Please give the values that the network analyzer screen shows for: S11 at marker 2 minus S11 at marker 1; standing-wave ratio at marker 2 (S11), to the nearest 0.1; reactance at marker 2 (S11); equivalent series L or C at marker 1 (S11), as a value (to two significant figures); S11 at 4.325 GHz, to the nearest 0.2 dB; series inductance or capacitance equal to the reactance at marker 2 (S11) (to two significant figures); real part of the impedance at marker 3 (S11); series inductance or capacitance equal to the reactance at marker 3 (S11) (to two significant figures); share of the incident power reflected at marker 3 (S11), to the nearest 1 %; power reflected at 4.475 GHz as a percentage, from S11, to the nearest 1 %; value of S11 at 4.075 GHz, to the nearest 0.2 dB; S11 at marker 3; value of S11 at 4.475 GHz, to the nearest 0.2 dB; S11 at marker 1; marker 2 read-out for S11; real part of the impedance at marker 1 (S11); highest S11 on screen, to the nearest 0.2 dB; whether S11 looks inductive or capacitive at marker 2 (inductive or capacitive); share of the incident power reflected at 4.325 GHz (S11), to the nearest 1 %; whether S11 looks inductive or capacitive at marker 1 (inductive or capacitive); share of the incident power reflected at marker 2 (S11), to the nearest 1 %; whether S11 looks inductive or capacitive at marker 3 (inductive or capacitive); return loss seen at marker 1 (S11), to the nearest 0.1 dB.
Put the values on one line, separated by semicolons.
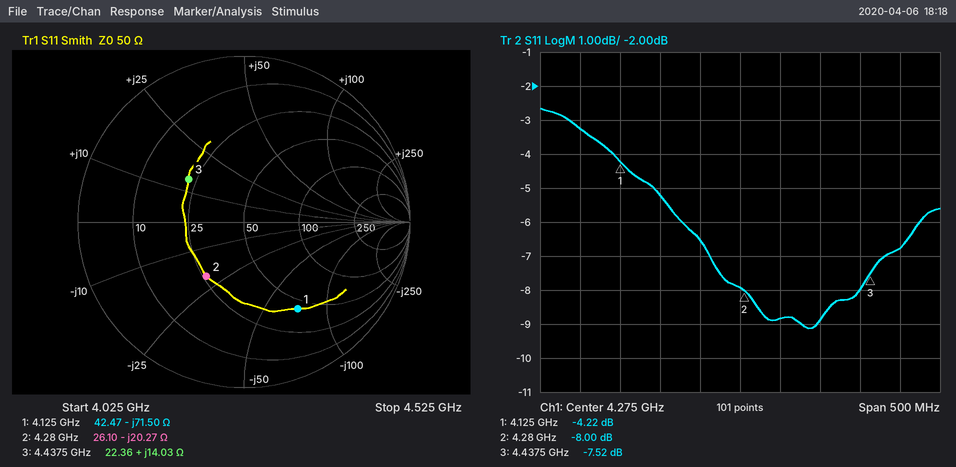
-3.78 dB; 2.3; -20.27 Ω; 540 fF; -8.8 dB; 1.8 pF; 22.36 Ω; 500 pH; 18 %; 21 %; -3.2 dB; -7.52 dB; -6.8 dB; -4.22 dB; -8.00 dB; 42.47 Ω; -2.6 dB; capacitive; 13 %; capacitive; 16 %; inductive; 4.2 dB
